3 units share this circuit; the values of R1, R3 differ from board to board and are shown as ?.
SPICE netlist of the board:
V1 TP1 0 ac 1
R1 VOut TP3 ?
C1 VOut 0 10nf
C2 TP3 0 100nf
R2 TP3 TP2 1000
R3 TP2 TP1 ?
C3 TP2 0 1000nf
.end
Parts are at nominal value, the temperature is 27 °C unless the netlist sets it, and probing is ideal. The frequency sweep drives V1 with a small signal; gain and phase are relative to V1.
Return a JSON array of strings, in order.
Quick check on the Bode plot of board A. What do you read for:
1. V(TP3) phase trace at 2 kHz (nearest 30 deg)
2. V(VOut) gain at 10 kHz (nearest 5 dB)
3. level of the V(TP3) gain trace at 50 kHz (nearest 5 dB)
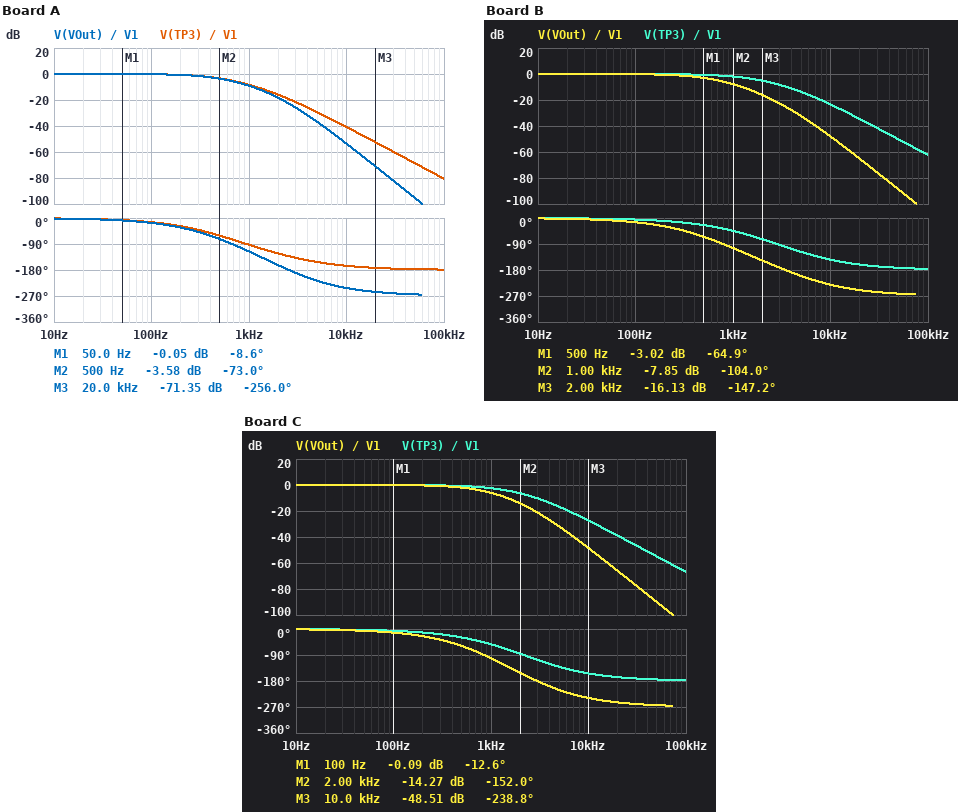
["-120 deg", "-55 dB", "-70 dB"]
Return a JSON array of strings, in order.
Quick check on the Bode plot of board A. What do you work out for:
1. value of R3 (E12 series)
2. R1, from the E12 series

["270 Ω", "6.8 kΩ"]
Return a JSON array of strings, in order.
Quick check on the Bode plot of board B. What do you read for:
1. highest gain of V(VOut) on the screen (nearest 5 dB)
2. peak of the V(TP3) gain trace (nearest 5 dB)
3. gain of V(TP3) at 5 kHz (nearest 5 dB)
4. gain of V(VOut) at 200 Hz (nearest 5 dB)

["0 dB", "0 dB", "-15 dB", "0 dB"]
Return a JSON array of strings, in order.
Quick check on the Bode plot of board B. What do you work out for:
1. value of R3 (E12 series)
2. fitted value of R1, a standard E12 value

["33 Ω", "27 kΩ"]
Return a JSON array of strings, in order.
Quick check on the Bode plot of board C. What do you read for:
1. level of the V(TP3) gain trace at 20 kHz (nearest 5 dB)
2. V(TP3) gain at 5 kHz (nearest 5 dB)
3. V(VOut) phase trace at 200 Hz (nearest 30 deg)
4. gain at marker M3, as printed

["-40 dB", "-15 dB", "-30 deg", "-48.51 dB"]
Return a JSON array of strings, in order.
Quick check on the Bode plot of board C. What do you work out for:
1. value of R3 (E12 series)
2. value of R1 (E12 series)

["56 Ω", "18 kΩ"]
